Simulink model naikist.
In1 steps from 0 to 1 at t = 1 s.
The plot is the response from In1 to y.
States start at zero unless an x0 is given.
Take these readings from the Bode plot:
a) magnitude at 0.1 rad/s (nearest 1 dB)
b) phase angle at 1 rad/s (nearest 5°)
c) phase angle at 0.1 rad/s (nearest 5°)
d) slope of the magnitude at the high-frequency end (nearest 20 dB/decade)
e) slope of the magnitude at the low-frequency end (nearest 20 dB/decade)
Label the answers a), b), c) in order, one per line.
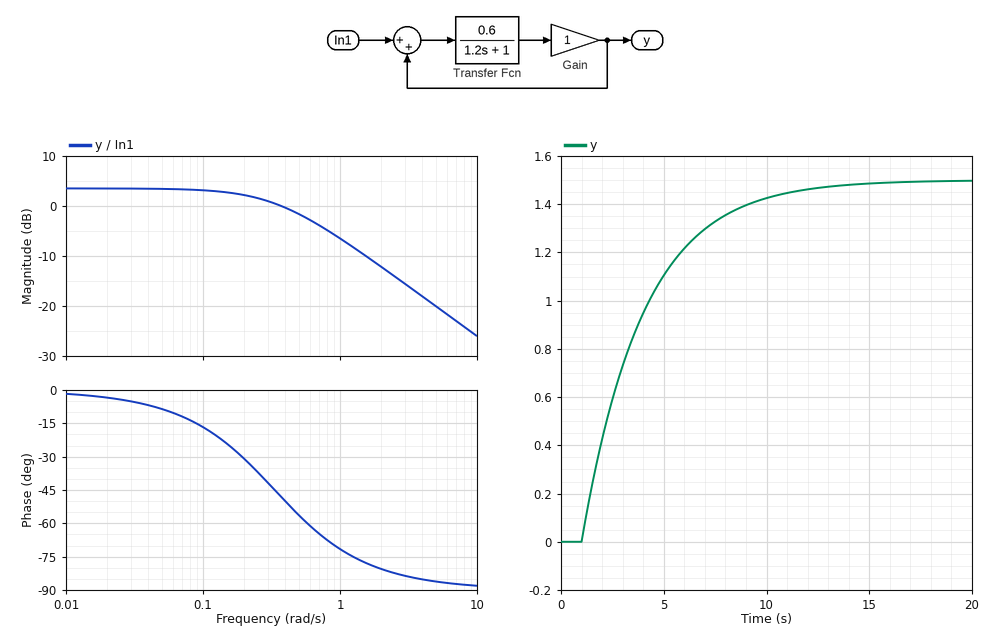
a) 3 dB
b) -70°
c) -15°
d) -20 dB/decade
e) 0 dB/decade
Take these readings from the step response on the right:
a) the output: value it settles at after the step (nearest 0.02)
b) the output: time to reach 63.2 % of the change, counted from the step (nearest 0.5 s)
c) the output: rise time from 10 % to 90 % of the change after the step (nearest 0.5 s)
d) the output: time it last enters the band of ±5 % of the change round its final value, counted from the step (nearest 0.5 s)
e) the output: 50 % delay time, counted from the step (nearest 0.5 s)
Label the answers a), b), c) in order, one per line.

a) 1.50
b) 3.0 s
c) 6.5 s
d) 9.0 s
e) 2.0 s
